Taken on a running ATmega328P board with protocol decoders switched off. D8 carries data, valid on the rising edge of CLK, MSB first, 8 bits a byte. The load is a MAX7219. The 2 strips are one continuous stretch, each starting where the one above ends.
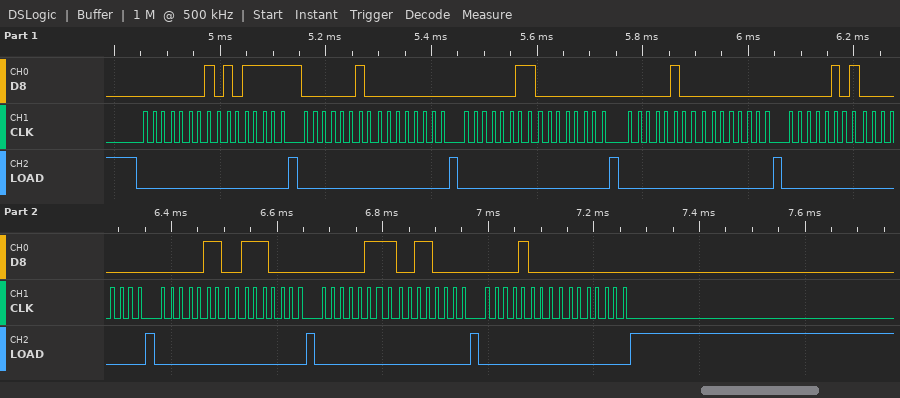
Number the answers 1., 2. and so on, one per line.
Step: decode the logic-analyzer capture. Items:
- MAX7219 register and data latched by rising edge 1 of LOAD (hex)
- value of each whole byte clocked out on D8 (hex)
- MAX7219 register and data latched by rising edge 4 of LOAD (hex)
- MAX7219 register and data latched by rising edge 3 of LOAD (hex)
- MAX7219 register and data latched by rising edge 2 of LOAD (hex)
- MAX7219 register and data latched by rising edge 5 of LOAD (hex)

1. register 0x1, data 0x5F
2. 01 5F 02 00 03 00 04 00 05 00 06 70 07 30 08 00
3. register 0x4, data 0x00
4. register 0x3, data 0x00
5. register 0x2, data 0x00
6. register 0x5, data 0x00
